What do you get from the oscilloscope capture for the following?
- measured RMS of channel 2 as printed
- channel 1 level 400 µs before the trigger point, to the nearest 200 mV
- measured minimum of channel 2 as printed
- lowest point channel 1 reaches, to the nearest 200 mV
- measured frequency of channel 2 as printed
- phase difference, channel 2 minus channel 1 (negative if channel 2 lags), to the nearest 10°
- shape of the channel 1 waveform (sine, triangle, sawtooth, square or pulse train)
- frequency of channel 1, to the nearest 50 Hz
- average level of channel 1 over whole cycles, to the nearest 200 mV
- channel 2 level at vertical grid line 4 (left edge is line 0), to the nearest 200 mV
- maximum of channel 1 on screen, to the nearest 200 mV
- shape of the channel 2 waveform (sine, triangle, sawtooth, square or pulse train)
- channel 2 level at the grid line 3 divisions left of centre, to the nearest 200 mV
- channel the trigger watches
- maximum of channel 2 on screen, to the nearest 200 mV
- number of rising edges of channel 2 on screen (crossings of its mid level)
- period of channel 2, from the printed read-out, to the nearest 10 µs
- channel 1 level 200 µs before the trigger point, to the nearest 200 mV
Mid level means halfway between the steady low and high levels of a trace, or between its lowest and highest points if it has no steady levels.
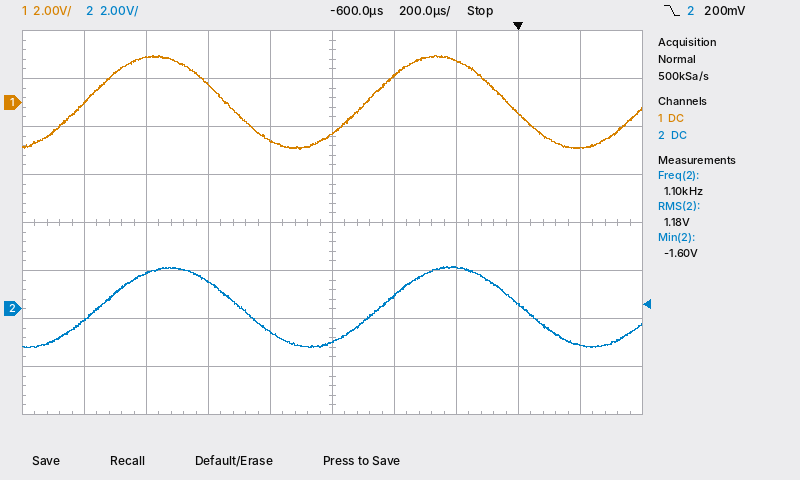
1.18 V
1.2 V
-1.60 V
-2.0 V
1.10 kHz
-20°
sine
1.10 kHz
0.0 V
-1.0 V
2.0 V
sine
1.4 V
channel 2
1.8 V
2
910 µs
1.8 V
